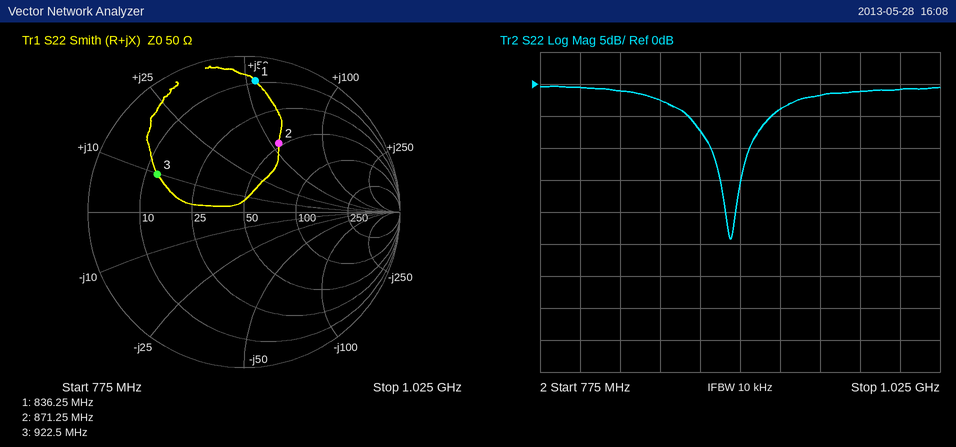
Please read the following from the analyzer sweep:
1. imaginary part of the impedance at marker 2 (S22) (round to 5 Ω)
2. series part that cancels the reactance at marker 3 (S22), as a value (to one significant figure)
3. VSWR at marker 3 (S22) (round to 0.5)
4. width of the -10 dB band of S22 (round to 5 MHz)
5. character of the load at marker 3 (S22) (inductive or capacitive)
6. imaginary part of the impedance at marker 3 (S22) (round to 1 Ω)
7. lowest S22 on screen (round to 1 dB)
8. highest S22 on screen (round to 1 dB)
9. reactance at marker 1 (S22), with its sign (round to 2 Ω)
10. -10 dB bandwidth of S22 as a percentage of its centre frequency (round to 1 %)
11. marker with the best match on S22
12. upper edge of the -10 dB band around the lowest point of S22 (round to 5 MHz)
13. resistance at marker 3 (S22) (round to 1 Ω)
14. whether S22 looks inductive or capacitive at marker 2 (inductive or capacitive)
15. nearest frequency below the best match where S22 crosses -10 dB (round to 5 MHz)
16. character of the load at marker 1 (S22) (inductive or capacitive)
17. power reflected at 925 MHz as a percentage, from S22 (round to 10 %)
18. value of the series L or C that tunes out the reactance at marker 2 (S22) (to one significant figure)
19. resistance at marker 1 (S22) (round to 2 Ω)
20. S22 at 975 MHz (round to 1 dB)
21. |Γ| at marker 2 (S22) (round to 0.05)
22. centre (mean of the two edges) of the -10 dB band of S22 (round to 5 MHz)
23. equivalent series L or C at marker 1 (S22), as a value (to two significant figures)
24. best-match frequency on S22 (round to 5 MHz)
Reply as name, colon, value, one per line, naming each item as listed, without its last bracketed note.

imaginary part of the impedance at marker 2 (S22): +55 Ω
series part that cancels the reactance at marker 3 (S22), as a value: 20 pF
VSWR at marker 3 (S22): 4.0
width of the -10 dB band of S22: 25 MHz
character of the load at marker 3 (S22): inductive
imaginary part of the impedance at marker 3 (S22): +10 Ω
lowest S22 on screen: -24 dB
highest S22 on screen: 0 dB
reactance at marker 1 (S22), with its sign: +54 Ω
-10 dB bandwidth of S22 as a percentage of its centre frequency: 3 %
marker with the best match on S22: marker 2
upper edge of the -10 dB band around the lowest point of S22: 905 MHz
resistance at marker 3 (S22): 13 Ω
whether S22 looks inductive or capacitive at marker 2: inductive
nearest frequency below the best match where S22 crosses -10 dB: 880 MHz
character of the load at marker 1 (S22): inductive
power reflected at 925 MHz as a percentage, from S22: 40 %
value of the series L or C that tunes out the reactance at marker 2 (S22): 3 pF
resistance at marker 1 (S22): 10 Ω
S22 at 975 MHz: -1 dB
|Γ| at marker 2 (S22): 0.50
centre (mean of the two edges) of the -10 dB band of S22: 895 MHz
equivalent series L or C at marker 1 (S22), as a value: 10 nH
best-match frequency on S22: 895 MHz
